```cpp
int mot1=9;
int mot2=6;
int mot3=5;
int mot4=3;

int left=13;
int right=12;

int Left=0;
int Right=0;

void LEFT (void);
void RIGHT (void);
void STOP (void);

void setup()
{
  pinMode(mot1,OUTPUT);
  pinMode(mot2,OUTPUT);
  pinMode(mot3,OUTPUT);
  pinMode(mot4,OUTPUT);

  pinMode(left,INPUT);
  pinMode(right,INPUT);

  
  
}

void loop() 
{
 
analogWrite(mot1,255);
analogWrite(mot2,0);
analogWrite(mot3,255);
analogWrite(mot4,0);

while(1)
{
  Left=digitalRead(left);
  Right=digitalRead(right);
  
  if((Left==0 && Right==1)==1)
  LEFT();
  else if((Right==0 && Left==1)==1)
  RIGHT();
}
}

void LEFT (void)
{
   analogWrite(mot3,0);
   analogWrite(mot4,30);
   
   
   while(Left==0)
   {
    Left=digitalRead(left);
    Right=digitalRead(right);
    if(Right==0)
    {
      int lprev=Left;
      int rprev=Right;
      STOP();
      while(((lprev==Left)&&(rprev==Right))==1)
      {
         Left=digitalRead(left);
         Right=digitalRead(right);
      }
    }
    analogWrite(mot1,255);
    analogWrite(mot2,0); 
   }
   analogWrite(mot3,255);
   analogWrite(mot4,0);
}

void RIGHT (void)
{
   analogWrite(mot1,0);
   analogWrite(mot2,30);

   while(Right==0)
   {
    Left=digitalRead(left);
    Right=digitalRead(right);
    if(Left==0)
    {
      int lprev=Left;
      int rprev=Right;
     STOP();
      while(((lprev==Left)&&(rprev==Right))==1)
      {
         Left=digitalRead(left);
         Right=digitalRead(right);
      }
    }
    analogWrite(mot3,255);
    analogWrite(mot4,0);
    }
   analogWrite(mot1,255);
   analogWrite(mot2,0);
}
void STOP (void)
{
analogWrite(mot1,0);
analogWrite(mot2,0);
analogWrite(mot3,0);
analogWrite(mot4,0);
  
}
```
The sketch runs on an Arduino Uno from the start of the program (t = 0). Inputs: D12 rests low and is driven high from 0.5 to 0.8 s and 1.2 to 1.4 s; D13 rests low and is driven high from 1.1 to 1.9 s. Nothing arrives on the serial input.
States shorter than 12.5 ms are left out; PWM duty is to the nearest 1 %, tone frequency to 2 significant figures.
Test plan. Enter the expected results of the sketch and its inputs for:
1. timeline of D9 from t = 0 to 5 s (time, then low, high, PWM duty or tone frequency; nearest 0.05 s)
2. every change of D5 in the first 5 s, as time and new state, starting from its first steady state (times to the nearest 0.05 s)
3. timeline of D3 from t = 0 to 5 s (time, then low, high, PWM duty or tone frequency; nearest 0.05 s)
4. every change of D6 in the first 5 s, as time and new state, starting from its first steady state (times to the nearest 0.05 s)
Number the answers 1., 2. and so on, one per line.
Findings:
1. 0 s high; 0.8 s low; 1.2 s high; 1.4 s low
2. 0 s high; 0.5 s low; 1.1 s high; 1.9 s low
3. 0 s low; 0.5 s PWM 12 %; 0.8 s low
4. 0 s low; 1.1 s PWM 12 %; 1.2 s low; 1.4 s PWM 12 %; 1.9 s low
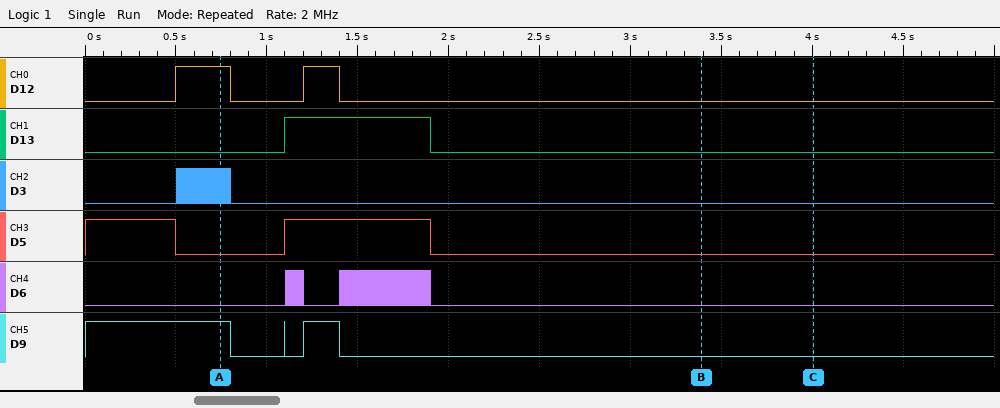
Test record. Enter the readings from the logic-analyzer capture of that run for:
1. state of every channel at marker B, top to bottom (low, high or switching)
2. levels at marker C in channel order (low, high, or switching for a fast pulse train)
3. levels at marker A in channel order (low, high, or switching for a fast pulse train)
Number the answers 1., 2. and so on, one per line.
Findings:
1. D12 low, D13 low, D3 low, D5 low, D6 low, D9 low
2. D12 low, D13 low, D3 low, D5 low, D6 low, D9 low
3. D12 high, D13 low, D3 switching, D5 low, D6 low, D9 high
